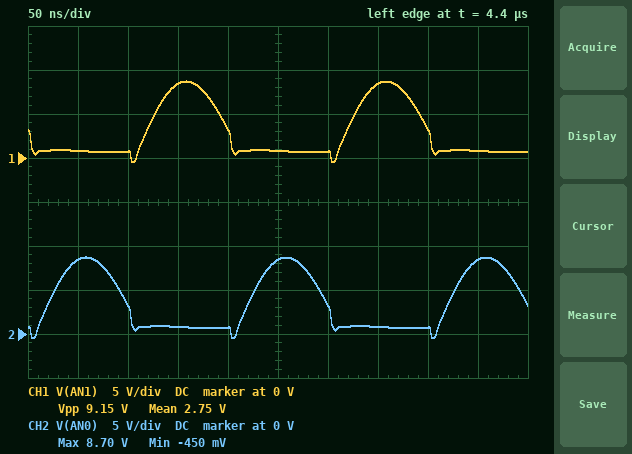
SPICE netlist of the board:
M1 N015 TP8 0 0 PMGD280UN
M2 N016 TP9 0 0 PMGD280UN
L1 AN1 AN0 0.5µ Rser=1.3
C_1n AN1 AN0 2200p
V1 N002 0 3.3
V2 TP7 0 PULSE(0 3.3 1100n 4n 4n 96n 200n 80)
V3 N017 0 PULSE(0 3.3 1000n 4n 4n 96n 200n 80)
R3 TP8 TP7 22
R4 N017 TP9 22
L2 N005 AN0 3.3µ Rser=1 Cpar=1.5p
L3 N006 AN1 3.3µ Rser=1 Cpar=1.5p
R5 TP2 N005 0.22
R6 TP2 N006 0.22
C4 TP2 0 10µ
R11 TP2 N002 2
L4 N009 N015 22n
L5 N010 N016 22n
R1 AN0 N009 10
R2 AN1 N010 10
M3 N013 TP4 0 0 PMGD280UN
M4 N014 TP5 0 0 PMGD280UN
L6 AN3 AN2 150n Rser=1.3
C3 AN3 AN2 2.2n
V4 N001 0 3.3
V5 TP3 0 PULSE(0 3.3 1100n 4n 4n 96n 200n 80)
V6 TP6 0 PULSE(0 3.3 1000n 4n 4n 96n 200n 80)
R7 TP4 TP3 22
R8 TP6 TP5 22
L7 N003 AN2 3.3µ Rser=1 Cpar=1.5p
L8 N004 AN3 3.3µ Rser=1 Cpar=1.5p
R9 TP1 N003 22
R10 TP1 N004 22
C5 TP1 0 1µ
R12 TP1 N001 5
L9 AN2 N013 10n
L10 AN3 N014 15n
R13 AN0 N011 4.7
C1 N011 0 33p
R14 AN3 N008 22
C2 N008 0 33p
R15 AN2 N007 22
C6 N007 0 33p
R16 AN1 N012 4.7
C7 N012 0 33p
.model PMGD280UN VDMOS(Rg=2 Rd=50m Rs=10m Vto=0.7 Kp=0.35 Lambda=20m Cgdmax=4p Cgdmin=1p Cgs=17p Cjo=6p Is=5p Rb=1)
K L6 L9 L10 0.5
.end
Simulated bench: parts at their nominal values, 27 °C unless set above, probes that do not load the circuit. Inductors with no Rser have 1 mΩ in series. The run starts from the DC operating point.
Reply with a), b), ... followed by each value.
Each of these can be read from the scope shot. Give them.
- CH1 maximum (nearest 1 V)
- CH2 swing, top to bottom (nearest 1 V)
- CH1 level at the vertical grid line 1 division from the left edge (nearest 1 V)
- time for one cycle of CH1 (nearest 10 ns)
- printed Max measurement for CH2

a) 9 V
b) 9 V
c) 1 V
d) 200 ns
e) 8.70 V
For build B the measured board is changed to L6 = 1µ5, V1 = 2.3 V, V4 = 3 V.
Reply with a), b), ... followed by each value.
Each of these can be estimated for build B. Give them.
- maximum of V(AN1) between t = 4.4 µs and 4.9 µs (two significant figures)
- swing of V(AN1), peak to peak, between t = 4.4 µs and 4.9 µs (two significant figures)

a) 6.1 V
b) 6.5 V
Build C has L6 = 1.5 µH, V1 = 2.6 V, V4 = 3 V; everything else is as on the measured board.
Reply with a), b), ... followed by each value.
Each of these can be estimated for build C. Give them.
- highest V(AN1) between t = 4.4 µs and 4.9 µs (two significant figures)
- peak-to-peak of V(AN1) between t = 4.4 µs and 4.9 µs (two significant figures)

a) 6.9 V
b) 7.3 V
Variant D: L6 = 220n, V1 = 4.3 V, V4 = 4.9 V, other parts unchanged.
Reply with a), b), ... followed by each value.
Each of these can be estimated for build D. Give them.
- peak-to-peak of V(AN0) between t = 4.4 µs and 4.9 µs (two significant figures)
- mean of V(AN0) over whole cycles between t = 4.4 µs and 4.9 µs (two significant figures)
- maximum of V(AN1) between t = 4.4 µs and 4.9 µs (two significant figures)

a) 12 V
b) 4.2 V
c) 11 V
